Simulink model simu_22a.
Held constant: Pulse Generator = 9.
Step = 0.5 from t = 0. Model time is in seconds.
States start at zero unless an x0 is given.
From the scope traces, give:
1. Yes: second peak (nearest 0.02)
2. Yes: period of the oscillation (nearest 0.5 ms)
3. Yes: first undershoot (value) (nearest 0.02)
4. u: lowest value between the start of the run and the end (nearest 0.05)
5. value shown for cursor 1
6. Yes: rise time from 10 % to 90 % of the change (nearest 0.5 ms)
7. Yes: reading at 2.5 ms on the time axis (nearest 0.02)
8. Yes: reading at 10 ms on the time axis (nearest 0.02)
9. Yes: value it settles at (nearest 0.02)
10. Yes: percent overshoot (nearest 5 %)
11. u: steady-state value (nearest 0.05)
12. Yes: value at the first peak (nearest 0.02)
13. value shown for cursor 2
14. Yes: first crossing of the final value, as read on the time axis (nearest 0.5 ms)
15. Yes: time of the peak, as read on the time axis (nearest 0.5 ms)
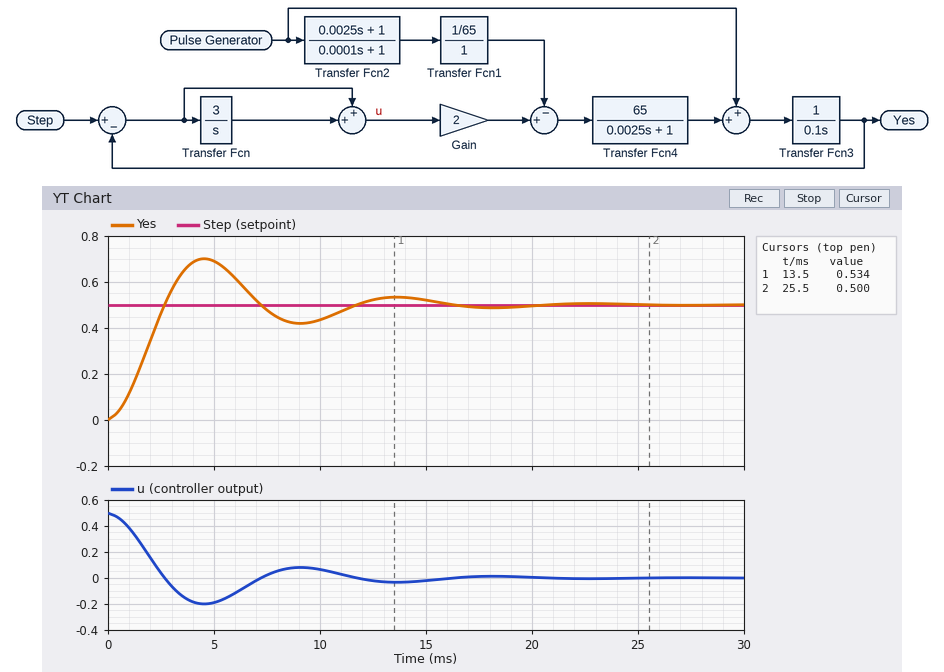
0.54
9.0 ms
0.42
-0.20
0.534
2.0 ms
0.46
0.44
0.50
40 %
0.00
0.70
0.500
2.5 ms
4.5 ms
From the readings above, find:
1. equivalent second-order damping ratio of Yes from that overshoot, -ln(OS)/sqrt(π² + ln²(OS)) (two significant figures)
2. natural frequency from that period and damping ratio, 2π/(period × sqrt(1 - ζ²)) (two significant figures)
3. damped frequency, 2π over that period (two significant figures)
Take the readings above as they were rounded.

0.28
0.73 rad/ms
0.70 rad/ms
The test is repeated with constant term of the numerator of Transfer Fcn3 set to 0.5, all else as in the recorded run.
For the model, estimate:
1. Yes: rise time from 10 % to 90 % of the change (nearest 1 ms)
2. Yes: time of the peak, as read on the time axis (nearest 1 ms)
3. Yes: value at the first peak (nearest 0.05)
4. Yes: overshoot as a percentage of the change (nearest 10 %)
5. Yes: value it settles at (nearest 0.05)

3 ms
7 ms
0.65
30 %
0.50
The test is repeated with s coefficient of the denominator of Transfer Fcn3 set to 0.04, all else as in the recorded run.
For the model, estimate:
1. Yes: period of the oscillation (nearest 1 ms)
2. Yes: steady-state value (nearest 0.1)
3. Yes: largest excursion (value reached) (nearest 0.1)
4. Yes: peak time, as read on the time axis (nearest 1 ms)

6 ms
0.5
0.8
3 ms
